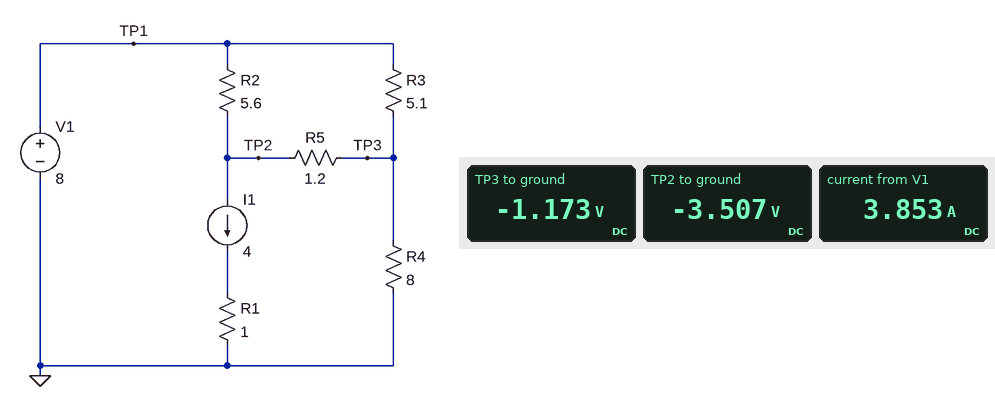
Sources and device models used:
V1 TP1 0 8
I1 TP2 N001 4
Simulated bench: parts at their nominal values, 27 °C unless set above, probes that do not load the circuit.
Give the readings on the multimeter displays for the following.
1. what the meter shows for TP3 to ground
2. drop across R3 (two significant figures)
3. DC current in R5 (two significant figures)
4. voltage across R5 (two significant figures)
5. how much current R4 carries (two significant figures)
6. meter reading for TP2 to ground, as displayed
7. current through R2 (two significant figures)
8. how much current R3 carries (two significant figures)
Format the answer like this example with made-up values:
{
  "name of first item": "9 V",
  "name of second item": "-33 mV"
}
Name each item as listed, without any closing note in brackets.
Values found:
{
  "what the meter shows for TP3 to ground": "-1.173 V",
  "drop across R3": "9.2 V",
  "DC current in R5": "1.9 A",
  "voltage across R5": "2.3 V",
  "how much current R4 carries": "150 mA",
  "meter reading for TP2 to ground, as displayed": "-3.507 V",
  "current through R2": "2.1 A",
  "how much current R3 carries": "1.8 A"
}
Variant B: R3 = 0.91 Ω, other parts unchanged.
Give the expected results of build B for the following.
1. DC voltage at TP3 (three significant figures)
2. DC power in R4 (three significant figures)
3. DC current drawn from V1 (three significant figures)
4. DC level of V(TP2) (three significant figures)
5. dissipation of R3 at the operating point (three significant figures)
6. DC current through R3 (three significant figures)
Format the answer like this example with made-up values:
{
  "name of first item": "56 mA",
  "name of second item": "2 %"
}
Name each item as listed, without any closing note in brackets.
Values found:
{
  "DC voltage at TP3": "4.87 V",
  "DC power in R4": "2.96 W",
  "DC current drawn from V1": "4.61 A",
  "DC level of V(TP2)": "1.47 V",
  "dissipation of R3 at the operating point": "10.8 W",
  "DC current through R3": "3.44 A"
}
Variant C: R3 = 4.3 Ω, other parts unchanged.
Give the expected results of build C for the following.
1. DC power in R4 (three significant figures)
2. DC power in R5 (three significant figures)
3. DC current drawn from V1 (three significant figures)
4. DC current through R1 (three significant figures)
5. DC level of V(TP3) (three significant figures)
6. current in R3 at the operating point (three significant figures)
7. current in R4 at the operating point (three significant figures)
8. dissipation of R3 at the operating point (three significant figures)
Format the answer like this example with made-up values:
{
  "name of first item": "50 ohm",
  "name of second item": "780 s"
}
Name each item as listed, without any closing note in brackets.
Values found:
{
  "DC power in R4": "32.5 mW",
  "DC power in R5": "5.01 W",
  "DC current drawn from V1": "3.94 A",
  "DC current through R1": "4.00 A",
  "DC level of V(TP3)": "-510 mV",
  "current in R3 at the operating point": "1.98 A",
  "current in R4 at the operating point": "63.7 mA",
  "dissipation of R3 at the operating point": "16.8 W"
}
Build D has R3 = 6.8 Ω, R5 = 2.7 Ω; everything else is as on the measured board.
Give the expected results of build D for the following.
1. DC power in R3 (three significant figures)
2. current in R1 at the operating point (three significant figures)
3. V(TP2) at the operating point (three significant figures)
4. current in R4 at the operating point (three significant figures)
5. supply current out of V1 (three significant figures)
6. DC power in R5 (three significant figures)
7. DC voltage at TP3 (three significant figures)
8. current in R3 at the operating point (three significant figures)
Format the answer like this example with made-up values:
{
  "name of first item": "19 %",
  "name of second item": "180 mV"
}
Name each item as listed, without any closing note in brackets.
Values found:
{
  "DC power in R3": "13.1 W",
  "current in R1 at the operating point": "4.00 A",
  "V(TP2) at the operating point": "-5.64 V",
  "current in R4 at the operating point": "178 mA",
  "supply current out of V1": "3.82 A",
  "DC power in R5": "6.60 W",
  "DC voltage at TP3": "-1.42 V",
  "current in R3 at the operating point": "1.39 A"
}
